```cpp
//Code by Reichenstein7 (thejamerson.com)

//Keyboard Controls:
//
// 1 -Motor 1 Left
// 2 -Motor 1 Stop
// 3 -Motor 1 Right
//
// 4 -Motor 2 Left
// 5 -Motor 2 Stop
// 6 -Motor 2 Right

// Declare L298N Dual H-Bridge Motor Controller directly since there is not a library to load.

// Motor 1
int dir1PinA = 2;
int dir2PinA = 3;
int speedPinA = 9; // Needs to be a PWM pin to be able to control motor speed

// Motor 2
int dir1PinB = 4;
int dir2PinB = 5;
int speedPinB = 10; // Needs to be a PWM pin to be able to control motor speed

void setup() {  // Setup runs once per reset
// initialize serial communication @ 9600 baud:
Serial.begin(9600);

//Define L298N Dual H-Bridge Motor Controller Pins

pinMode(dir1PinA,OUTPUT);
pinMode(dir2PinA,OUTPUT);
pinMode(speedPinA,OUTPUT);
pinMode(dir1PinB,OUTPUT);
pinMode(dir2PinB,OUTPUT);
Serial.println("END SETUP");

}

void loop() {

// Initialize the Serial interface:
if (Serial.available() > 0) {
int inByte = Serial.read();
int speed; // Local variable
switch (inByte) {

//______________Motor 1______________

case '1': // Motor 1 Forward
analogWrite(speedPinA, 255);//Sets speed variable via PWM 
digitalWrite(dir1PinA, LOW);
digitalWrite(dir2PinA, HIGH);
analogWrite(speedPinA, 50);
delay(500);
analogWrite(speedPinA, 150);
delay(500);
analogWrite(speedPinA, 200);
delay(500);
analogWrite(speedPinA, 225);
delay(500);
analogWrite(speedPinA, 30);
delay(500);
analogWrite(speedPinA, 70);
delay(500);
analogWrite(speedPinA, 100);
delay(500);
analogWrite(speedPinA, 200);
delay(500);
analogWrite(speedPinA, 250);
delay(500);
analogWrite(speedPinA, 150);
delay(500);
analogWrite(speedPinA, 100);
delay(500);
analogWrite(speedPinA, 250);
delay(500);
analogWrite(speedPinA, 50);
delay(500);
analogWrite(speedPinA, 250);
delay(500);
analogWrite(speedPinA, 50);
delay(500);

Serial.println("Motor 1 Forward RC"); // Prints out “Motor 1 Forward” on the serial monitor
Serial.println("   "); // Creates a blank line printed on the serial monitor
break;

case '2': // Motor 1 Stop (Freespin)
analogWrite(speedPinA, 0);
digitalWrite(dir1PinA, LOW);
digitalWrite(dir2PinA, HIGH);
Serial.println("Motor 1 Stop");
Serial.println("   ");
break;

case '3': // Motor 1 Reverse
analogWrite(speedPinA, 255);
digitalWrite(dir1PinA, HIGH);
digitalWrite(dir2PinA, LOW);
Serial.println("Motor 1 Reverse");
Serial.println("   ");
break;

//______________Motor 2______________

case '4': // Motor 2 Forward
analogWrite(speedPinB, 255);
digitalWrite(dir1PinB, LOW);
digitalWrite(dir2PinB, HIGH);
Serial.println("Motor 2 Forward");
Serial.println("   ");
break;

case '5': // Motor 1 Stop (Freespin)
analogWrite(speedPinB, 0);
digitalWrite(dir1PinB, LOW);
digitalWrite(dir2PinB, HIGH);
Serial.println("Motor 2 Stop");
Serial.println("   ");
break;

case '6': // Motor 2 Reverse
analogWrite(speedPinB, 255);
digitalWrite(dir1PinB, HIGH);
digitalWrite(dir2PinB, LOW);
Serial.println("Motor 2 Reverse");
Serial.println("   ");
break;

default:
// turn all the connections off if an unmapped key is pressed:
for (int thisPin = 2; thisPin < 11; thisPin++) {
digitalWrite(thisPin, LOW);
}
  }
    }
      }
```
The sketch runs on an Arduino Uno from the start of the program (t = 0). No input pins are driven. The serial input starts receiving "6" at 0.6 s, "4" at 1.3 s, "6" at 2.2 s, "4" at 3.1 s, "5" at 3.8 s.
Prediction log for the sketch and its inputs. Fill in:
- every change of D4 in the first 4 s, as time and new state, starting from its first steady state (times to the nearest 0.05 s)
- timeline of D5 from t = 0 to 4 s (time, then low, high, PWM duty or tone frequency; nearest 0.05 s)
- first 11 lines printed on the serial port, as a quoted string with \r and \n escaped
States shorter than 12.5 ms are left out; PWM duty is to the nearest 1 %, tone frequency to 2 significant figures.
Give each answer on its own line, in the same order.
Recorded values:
0 s low; 0.6 s high; 1.3 s low; 2.2 s high; 3.1 s low
0 s low; 1.3 s high; 2.2 s low; 3.1 s high
"END SETUP\r\nMotor 2 Reverse\r\n   \r\nMotor 2 Forward\r\n   \r\nMotor 2 Reverse\r\n   \r\nMotor 2 Forward\r\n   \r\nMotor 2 Stop\r\n   \r\n"
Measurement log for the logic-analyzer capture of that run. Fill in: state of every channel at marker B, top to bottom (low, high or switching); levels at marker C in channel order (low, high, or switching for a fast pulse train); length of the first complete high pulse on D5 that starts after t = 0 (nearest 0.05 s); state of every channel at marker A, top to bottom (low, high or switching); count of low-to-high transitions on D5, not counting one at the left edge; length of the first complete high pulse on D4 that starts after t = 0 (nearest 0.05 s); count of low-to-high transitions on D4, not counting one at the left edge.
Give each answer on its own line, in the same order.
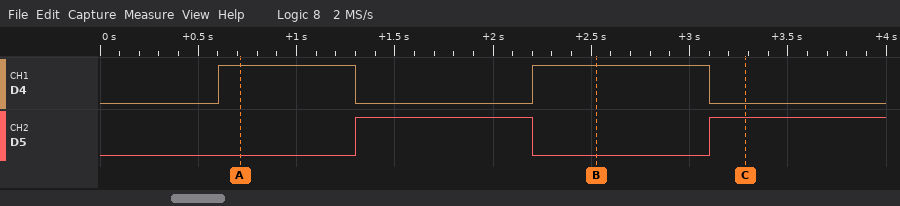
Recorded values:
D4 high, D5 low
D4 low, D5 high
0.90 s
D4 high, D5 low
2
0.70 s
2
